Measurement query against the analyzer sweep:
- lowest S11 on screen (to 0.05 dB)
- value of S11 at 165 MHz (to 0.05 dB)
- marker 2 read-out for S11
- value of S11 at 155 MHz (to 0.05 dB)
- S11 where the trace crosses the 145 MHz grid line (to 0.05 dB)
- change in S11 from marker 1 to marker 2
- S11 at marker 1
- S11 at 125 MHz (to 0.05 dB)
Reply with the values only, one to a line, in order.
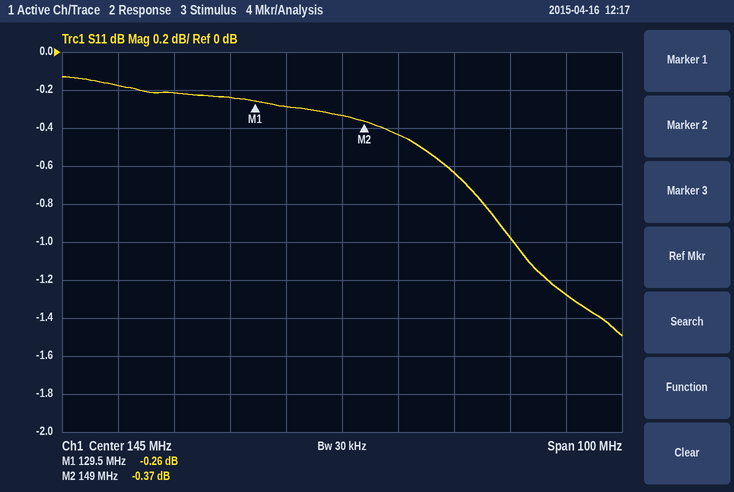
-1.50 dB
-0.65 dB
-0.37 dB
-0.45 dB
-0.35 dB
-0.11 dB
-0.26 dB
-0.25 dB
